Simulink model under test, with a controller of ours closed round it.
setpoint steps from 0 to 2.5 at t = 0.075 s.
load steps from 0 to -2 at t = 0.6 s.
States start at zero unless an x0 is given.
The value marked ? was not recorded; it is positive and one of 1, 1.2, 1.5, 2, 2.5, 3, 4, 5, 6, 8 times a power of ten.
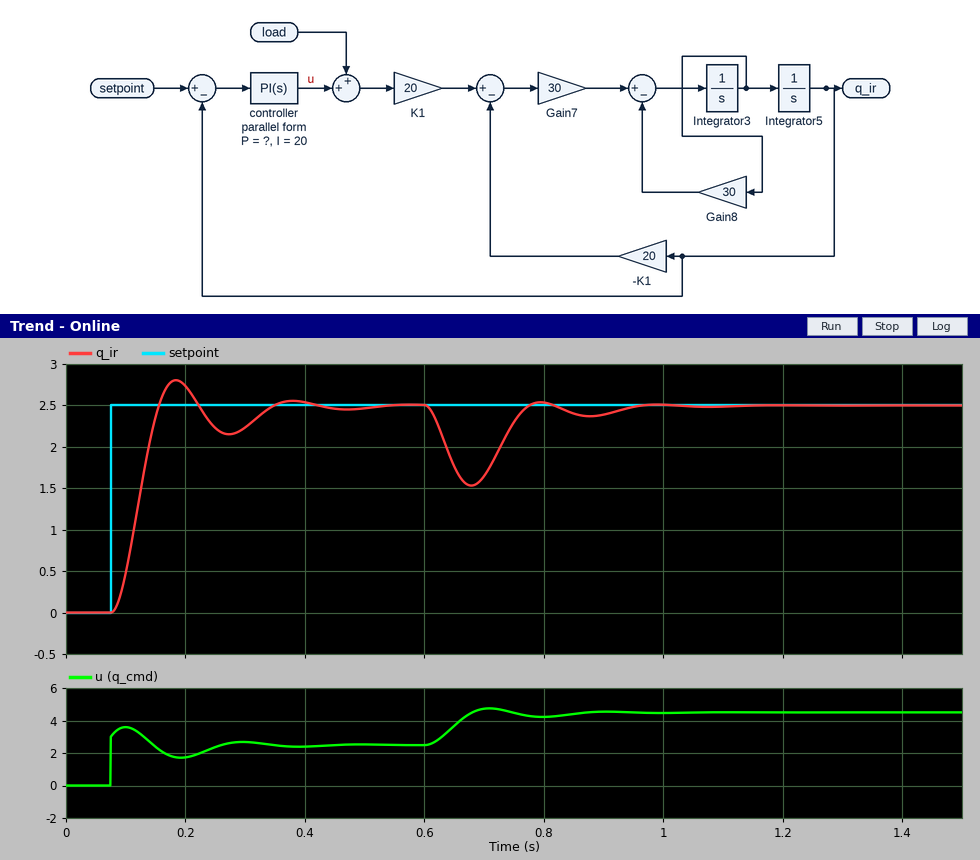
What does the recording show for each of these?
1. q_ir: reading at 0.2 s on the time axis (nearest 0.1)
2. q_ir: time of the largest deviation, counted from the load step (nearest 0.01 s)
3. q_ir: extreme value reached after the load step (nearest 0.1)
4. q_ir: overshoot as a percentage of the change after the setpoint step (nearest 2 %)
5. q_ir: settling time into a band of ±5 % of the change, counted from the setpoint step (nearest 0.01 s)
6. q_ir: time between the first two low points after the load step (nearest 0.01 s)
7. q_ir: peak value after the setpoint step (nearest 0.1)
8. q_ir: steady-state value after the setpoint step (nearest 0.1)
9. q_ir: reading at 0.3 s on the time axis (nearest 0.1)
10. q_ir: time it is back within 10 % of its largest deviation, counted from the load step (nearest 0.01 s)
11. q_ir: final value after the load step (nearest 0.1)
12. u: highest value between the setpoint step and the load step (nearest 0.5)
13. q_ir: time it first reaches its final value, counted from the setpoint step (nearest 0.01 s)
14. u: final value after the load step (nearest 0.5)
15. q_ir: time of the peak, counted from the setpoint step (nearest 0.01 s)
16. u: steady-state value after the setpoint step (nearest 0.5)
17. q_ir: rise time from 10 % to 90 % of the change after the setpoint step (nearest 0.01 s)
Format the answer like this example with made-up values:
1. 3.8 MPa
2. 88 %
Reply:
1. 2.7
2. 0.08 s
3. 1.5
4. 12 %
5. 0.25 s
6. 0.20 s
7. 2.8
8. 2.5
9. 2.2
10. 0.31 s
11. 2.5
12. 3.5
13. 0.08 s
14. 4.5
15. 0.11 s
16. 2.5
17. 0.05 s
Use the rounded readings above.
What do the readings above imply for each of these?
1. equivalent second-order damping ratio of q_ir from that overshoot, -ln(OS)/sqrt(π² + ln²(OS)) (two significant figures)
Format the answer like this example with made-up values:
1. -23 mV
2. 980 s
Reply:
1. 0.56
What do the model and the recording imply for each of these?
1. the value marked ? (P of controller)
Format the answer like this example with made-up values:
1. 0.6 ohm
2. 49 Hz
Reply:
1. 1.2
